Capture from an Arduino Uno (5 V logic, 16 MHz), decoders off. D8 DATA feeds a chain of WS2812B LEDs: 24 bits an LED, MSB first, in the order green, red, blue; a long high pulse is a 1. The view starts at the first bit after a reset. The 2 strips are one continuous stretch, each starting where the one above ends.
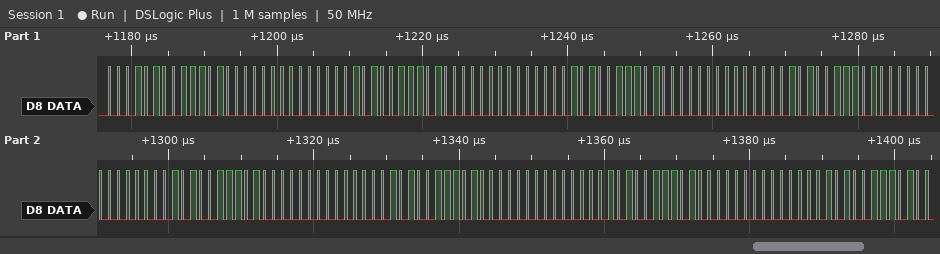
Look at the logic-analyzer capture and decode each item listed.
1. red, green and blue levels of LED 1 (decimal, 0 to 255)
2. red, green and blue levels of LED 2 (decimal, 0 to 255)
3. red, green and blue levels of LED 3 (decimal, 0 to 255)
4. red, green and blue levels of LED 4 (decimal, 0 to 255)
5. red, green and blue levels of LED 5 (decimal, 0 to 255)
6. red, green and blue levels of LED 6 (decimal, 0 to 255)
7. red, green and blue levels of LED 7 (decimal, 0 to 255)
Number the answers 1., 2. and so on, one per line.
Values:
1. 232, 20, 0
2. 232, 20, 0
3. 232, 20, 0
4. 232, 20, 0
5. 232, 20, 0
6. 232, 20, 0
7. 232, 20, 0
